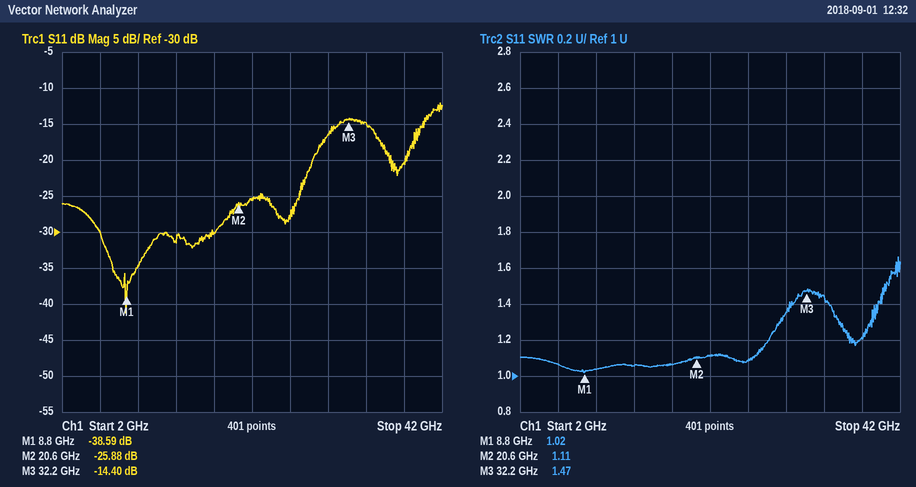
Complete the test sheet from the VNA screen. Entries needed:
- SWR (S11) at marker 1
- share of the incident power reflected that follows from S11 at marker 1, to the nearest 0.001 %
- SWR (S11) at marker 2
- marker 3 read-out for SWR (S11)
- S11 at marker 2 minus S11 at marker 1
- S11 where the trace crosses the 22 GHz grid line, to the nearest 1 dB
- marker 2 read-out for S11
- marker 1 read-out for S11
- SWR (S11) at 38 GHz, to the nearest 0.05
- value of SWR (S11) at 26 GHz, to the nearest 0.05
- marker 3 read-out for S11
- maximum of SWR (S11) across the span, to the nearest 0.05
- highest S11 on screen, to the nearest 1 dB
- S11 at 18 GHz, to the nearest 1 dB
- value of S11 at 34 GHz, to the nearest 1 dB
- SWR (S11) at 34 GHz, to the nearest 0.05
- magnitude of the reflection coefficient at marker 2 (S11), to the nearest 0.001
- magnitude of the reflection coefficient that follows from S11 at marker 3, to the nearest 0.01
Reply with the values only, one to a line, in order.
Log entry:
1.02
0.014 %
1.11
1.47
12.71 dB
-25 dB
-25.88 dB
-38.59 dB
1.20
1.10
-14.40 dB
1.65
-12 dB
-30 dB
-15 dB
1.45
0.051
0.19
